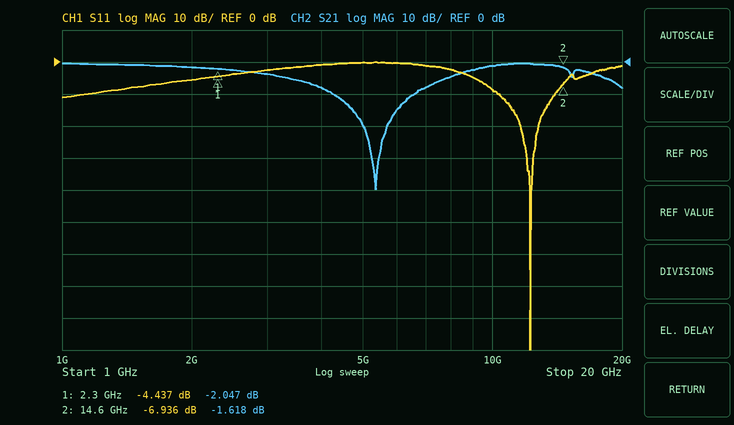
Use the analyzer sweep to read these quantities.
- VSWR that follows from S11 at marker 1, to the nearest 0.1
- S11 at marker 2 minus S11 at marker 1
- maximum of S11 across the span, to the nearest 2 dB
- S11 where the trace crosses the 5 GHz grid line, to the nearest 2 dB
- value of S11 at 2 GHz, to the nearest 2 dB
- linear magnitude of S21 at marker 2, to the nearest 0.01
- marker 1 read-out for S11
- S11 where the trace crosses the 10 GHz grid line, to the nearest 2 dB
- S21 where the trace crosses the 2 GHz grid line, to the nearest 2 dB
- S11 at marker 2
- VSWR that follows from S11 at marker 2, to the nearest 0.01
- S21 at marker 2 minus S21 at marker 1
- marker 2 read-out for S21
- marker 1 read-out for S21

4.0
-2.499 dB
0 dB
0 dB
-6 dB
0.83
-4.437 dB
-8 dB
-2 dB
-6.936 dB
2.64
0.429 dB
-1.618 dB
-2.047 dB
